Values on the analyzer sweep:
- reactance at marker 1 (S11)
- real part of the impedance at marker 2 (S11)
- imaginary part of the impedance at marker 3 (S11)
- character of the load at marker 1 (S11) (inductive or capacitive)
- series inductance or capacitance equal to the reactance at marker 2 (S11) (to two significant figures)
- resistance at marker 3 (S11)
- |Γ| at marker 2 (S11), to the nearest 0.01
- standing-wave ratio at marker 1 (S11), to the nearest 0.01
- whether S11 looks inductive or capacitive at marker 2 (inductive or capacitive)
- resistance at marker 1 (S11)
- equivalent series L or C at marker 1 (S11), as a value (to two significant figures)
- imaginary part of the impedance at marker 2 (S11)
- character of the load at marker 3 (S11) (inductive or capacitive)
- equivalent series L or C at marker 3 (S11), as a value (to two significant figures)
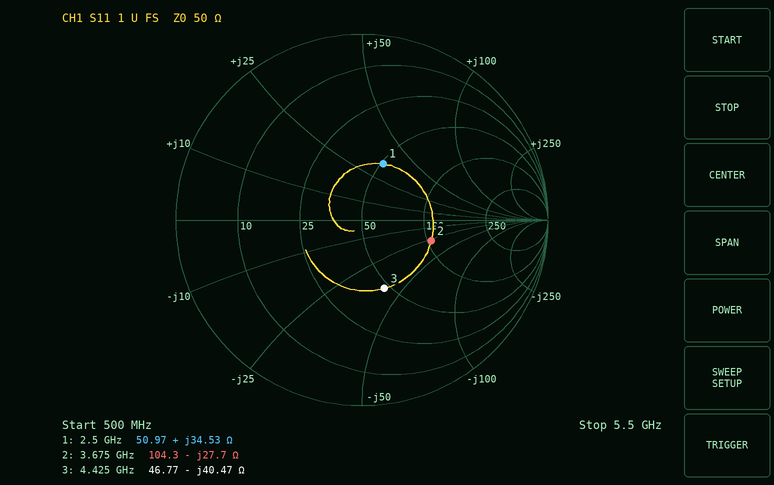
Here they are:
+34.53 Ω
104.3 Ω
-40.47 Ω
inductive
1.6 pF
46.77 Ω
0.39
1.96
capacitive
50.97 Ω
2.2 nH
-27.7 Ω
capacitive
890 fF
